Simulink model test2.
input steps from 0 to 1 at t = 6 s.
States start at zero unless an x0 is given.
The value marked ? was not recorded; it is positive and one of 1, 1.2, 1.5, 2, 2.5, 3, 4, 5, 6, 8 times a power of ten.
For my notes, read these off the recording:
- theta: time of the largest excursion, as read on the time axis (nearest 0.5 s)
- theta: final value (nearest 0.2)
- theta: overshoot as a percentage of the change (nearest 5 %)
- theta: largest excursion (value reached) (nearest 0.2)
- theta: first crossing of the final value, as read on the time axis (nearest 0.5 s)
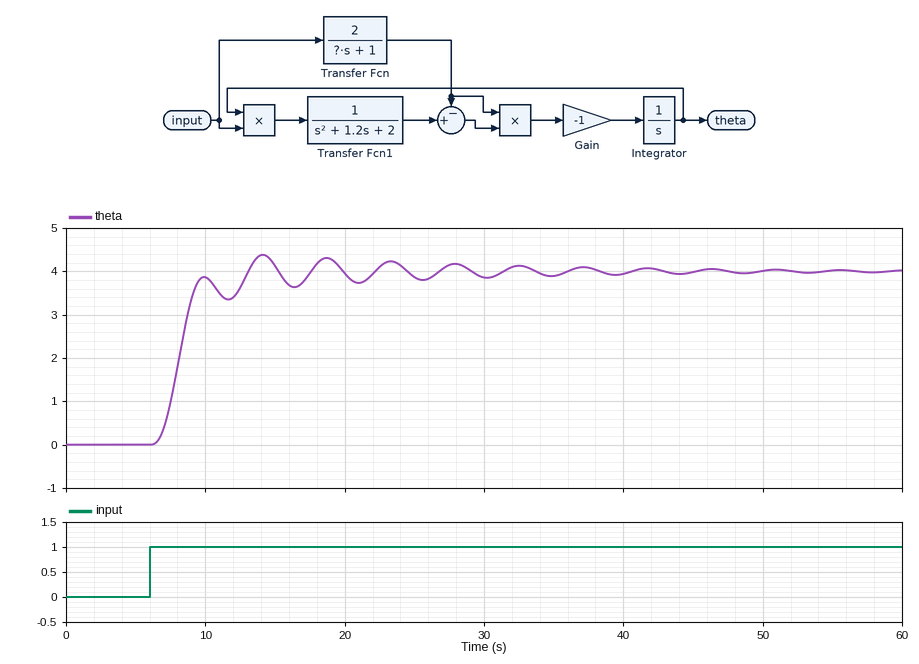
14.0 s
4.0
10 %
4.4
13.0 s
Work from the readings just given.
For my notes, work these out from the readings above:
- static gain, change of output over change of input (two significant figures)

4.0
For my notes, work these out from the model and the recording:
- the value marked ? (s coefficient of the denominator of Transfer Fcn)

1.5
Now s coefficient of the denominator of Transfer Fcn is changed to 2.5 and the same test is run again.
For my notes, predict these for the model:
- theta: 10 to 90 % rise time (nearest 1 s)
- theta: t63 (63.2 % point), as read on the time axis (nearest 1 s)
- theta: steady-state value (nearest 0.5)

6 s
9 s
4.0
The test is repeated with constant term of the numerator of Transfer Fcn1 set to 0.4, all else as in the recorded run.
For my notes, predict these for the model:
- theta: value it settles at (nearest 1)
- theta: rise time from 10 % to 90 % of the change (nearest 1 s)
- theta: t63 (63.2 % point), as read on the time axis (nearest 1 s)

10
6 s
10 s
